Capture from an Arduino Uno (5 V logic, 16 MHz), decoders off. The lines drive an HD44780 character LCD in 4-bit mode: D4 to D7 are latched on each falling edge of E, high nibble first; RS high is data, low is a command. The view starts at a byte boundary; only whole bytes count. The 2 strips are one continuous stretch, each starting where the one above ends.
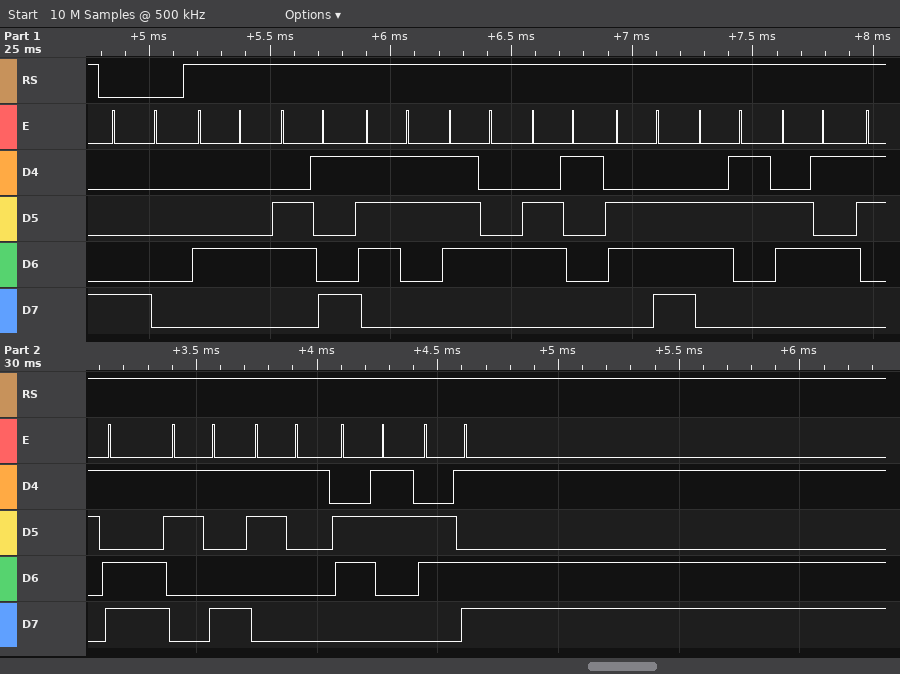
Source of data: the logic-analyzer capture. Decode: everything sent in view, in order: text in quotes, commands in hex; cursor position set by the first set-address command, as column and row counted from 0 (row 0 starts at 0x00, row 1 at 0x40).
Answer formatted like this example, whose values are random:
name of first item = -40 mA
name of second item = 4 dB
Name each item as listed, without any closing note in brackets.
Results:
everything sent in view, in order: text in quotes, commands in hex = 0x80 "Distance=91cm"
cursor position set by the first set-address command, as column and row counted from 0 = column 0, row 0
